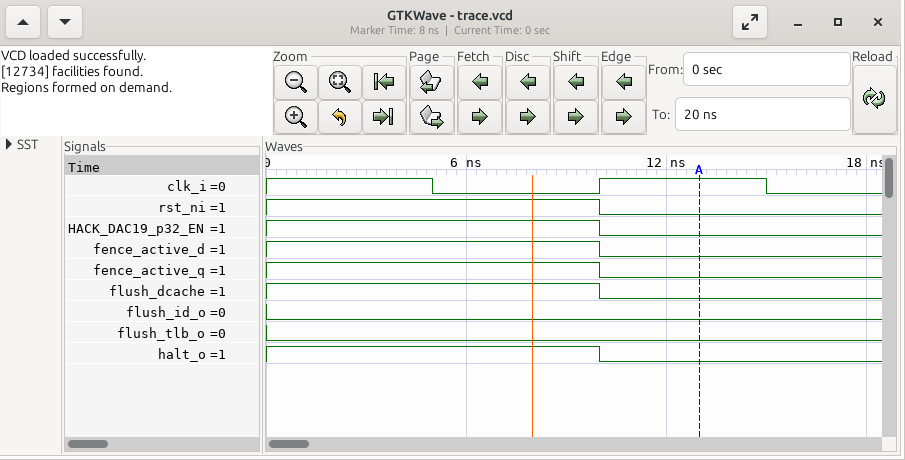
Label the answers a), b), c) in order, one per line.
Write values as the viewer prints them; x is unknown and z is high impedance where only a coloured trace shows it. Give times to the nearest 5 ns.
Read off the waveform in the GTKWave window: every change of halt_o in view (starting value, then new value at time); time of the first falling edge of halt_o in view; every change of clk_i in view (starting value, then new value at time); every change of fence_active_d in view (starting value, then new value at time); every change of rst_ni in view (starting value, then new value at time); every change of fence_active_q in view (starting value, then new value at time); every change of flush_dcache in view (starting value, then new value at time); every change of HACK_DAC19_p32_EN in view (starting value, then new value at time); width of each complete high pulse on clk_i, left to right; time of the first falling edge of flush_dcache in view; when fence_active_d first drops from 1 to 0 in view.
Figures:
a) 1, 0 at 10 ns
b) 10 ns
c) 1, 0 at 5 ns, 1 at 10 ns, 0 at 15 ns
d) 1, 0 at 10 ns
e) 1, 0 at 10 ns
f) 1, 0 at 10 ns
g) 1, 0 at 10 ns
h) 1, 0 at 10 ns
i) 5 ns
j) 10 ns
k) 10 ns
